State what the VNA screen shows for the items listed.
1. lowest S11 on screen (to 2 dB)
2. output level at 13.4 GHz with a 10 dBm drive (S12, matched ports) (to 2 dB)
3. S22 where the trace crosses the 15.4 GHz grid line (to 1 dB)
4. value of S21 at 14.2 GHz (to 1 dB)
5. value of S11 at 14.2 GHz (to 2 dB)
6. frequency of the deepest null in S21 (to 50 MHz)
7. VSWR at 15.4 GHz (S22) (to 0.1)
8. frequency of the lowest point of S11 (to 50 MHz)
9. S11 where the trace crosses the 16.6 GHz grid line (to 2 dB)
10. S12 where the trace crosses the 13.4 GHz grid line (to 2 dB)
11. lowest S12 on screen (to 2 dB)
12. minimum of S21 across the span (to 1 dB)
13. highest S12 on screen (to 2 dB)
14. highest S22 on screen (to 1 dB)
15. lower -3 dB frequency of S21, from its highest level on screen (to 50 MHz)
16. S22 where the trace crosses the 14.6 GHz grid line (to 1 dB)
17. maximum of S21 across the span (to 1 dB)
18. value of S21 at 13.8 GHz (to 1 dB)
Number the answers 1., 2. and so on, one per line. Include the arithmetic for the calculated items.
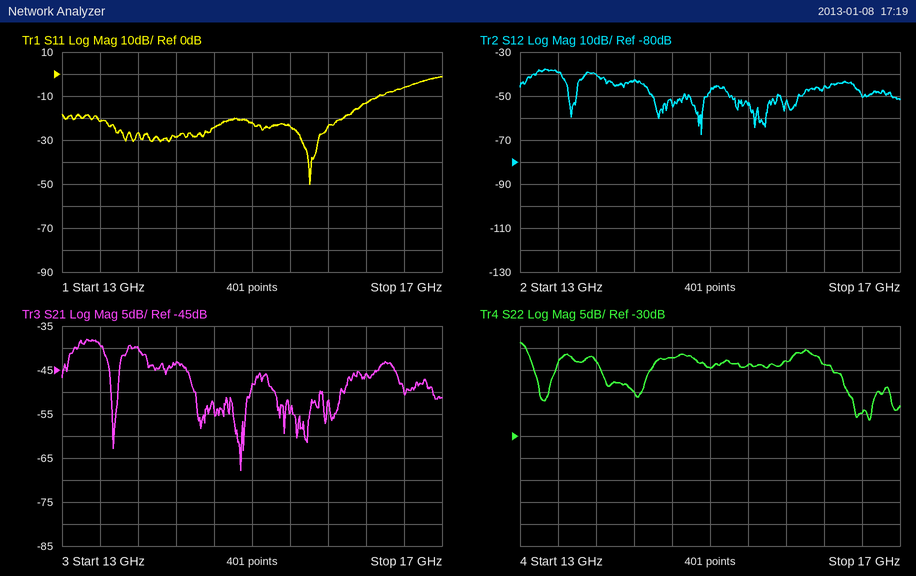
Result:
1. -50 dB
2. 10 dBm + (-40 dB) = -30 dBm
3. -14 dB
4. -43 dB
5. -28 dB
6. 14.90 GHz
7. |Γ| = 10^(-14/20) = 0.1995; VSWR = (1 + 0.1995)/(1 − 0.1995) ≈ 1.5
8. 15.60 GHz
9. -6 dB
10. -40 dB
11. -68 dB
12. -68 dB
13. -38 dB
14. -9 dB
15. 13.10 GHz
16. -12 dB
17. -38 dB
18. -40 dB
